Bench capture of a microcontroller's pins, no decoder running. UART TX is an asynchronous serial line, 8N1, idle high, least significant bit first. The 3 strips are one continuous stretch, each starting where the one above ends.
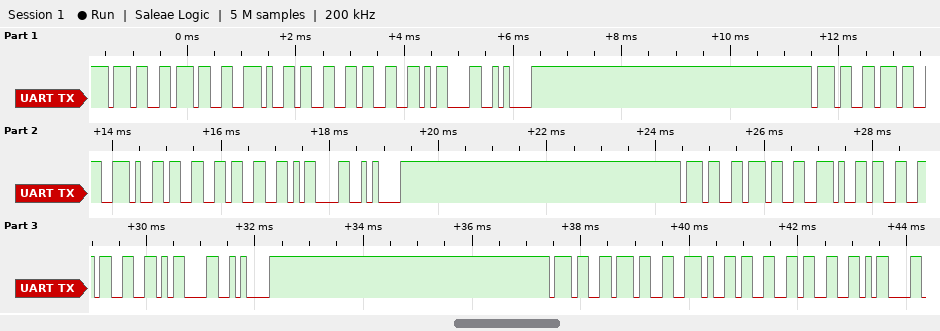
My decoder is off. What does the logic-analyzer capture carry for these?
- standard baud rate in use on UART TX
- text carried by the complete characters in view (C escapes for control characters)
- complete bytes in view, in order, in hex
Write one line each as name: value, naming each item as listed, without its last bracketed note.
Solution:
standard baud rate in use on UART TX: 9600 baud
text carried by the complete characters in view: "77.33\r\n77.33\r\n77.33\r\n77.33\r"
complete bytes in view, in order, in hex: 37 37 2E 33 33 0D 0A 37 37 2E 33 33 0D 0A 37 37 2E 33 33 0D 0A 37 37 2E 33 33 0D
